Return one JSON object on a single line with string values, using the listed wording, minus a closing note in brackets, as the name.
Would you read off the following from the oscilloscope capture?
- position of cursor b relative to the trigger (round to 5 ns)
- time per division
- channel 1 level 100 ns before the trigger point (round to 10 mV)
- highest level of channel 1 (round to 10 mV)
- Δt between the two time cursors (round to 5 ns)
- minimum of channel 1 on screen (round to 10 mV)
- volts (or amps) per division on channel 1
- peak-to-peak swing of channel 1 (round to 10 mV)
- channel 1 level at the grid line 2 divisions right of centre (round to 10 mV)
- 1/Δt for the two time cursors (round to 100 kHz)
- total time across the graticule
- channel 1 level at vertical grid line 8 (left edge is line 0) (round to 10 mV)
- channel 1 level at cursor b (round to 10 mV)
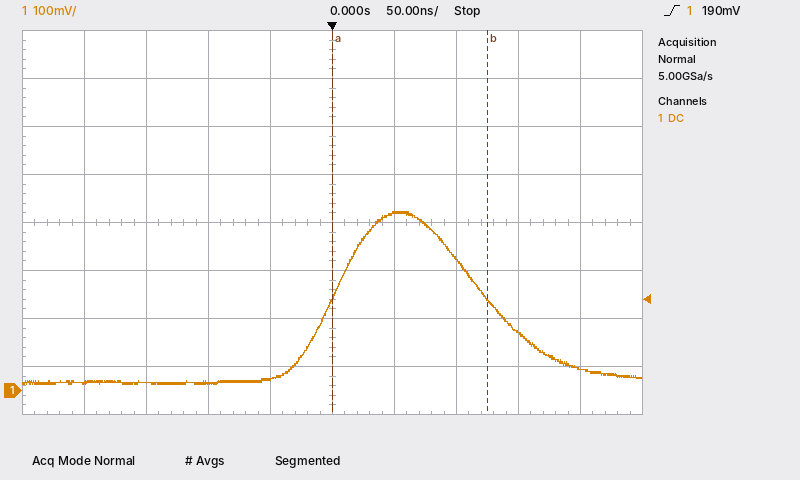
{"position of cursor b relative to the trigger": "+125 ns", "time per division": "50 ns", "channel 1 level 100 ns before the trigger point": "20 mV", "highest level of channel 1": "370 mV", "Δt between the two time cursors": "125 ns", "minimum of channel 1 on screen": "10 mV", "volts (or amps) per division on channel 1": "100 mV", "peak-to-peak swing of channel 1": "360 mV", "channel 1 level at the grid line 2 divisions right of centre": "270 mV", "1/Δt for the two time cursors": "8.0 MHz", "total time across the graticule": "500 ns", "channel 1 level at vertical grid line 8 (left edge is line 0)": "120 mV", "channel 1 level at cursor b": "190 mV"}
